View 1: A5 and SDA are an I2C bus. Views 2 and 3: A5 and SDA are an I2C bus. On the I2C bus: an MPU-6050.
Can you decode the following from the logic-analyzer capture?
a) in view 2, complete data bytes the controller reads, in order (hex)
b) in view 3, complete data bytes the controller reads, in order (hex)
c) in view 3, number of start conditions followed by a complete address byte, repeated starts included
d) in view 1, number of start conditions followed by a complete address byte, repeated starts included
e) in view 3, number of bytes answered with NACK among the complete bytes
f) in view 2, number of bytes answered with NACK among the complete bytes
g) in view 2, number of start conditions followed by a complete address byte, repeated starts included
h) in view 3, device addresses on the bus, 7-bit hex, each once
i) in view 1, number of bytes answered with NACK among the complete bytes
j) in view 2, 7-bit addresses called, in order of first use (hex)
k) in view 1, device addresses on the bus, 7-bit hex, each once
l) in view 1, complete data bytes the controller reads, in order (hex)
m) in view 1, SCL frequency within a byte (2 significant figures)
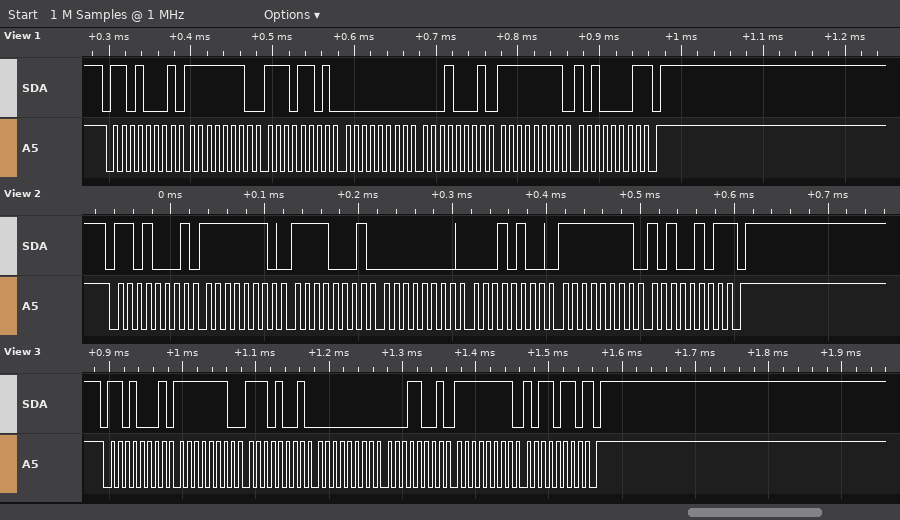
FE F1 00 14 FF A5
FE E9 00 19 FF B6
1
1
1
1
1
0x68
1
0x68
0x68
FE ED 00 11 FF A1
100 kHz
